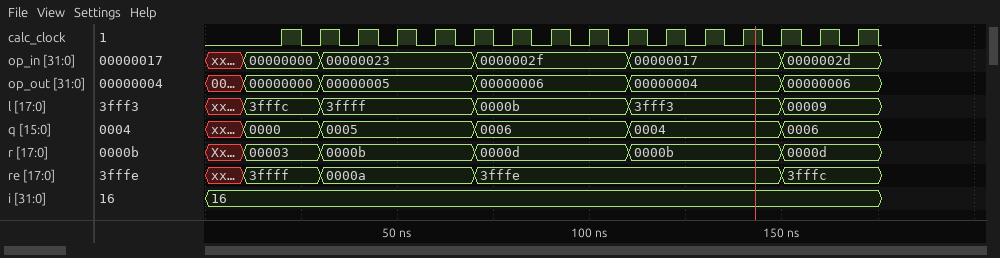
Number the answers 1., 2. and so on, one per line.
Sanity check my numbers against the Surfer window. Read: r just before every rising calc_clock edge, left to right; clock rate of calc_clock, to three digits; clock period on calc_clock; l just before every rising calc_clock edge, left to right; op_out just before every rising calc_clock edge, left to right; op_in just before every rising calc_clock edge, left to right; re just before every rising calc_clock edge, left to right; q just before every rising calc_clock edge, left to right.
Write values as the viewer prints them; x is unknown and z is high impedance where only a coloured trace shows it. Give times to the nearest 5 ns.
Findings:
1. 00003, 00003, 0000b, 0000b, 0000b, 0000b, 0000d, 0000d, 0000d, 0000d, 0000b, 0000b, 0000b, 0000b, 0000d, 0000d
2. 100 MHz
3. 10 ns
4. 3fffc, 3fffc, 3ffff, 3ffff, 3ffff, 3ffff, 0000b, 0000b, 0000b, 0000b, 3fff3, 3fff3, 3fff3, 3fff3, 00009, 00009
5. 00000000, 00000000, 00000005, 00000005, 00000005, 00000005, 00000006, 00000006, 00000006, 00000006, 00000004, 00000004, 00000004, 00000004, 00000006, 00000006
6. 00000000, 00000000, 00000023, 00000023, 00000023, 00000023, 0000002f, 0000002f, 0000002f, 0000002f, 00000017, 00000017, 00000017, 00000017, 0000002d, 0000002d
7. 3ffff, 3ffff, 0000a, 0000a, 0000a, 0000a, 3fffe, 3fffe, 3fffe, 3fffe, 3fffe, 3fffe, 3fffe, 3fffe, 3fffc, 3fffc
8. 0000, 0000, 0005, 0005, 0005, 0005, 0006, 0006, 0006, 0006, 0004, 0004, 0004, 0004, 0006, 0006
